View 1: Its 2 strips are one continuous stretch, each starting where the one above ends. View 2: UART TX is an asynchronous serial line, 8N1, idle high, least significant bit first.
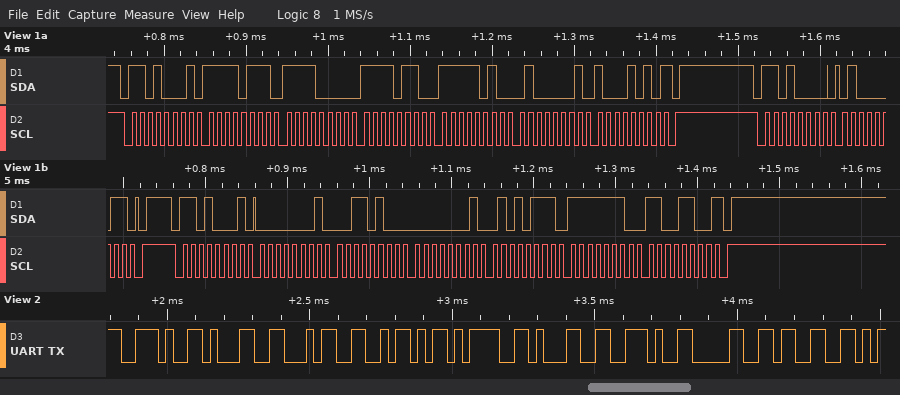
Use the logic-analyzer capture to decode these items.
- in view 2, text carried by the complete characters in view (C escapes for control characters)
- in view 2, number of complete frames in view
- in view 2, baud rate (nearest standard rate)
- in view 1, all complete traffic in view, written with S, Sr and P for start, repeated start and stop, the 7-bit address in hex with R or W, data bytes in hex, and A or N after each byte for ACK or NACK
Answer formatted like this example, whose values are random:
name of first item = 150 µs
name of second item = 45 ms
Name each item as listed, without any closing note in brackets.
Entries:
in view 2, text carried by the complete characters in view = ".14Z=1.03"
in view 2, number of complete frames in view = 9
in view 2, baud rate = 38400 baud
in view 1, all complete traffic in view, written with S, Sr and P for start, repeated start and stop, the 7-bit address in hex with R or W, data bytes in hex, and A or N after each byte for ACK or NACK = S 68R A F7 A F0 A F6 A FA A 41 A 8A N P S 68W A 43 A P S 68R A 01 A 34 A 01 A 57 A FE A CC N P
